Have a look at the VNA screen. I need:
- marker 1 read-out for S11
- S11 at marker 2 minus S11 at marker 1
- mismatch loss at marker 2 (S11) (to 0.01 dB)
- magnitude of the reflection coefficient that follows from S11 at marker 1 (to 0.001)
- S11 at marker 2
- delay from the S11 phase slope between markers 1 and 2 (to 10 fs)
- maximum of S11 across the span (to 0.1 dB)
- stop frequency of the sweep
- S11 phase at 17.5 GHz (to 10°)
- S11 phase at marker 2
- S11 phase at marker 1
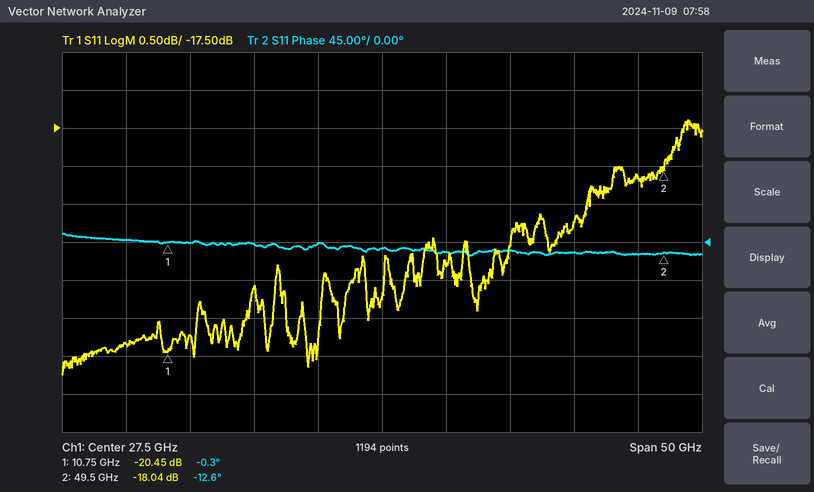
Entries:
-20.45 dB
2.41 dB
0.07 dB
0.095
-18.04 dB
880 fs
-17.4 dB
52.5 GHz
0°
-12.6°
-0.3°
